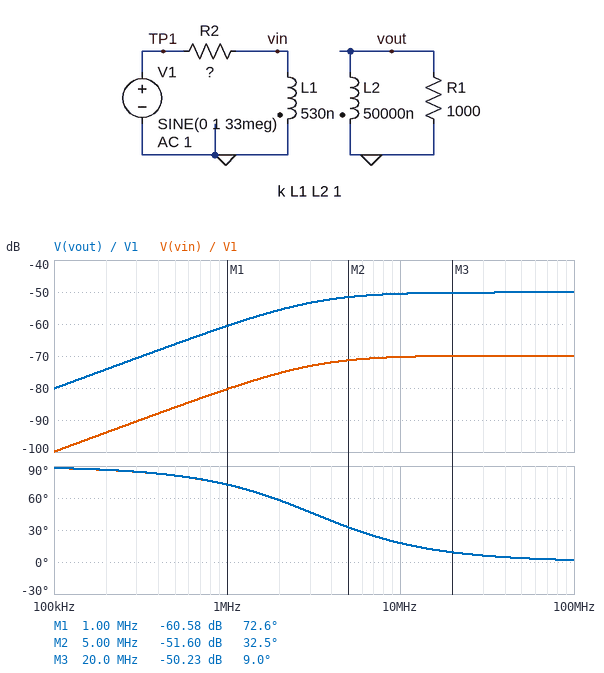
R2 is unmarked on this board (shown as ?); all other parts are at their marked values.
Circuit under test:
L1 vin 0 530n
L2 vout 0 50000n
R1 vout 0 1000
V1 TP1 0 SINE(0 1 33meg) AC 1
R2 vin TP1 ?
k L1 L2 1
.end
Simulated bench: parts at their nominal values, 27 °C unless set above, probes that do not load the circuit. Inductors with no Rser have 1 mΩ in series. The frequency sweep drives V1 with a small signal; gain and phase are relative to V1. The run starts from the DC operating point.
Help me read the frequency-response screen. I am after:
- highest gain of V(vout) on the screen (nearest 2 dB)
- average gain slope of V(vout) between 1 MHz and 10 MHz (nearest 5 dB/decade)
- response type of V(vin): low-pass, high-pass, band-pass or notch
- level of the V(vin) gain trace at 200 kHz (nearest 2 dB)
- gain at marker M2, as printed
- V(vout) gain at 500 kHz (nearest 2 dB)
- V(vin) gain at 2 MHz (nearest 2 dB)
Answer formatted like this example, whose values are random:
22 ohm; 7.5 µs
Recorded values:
-50 dB; 10 dB/decade; high-pass; -94 dB; -51.60 dB; -66 dB; -76 dB
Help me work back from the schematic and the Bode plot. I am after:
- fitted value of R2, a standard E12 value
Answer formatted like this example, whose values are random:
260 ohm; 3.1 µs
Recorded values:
33 kΩ
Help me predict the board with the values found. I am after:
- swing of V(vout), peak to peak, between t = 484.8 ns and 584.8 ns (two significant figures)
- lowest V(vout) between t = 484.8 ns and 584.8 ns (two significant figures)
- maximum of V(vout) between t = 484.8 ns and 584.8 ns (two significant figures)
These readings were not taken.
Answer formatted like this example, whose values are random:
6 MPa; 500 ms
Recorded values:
6.2 mV; -3.1 mV; 3.1 mV
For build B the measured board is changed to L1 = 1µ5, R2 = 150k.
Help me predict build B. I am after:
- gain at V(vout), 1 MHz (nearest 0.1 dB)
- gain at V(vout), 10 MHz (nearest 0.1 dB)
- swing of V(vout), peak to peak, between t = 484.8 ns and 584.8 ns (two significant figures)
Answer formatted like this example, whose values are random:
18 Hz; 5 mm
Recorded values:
-69.2 dB; -59.2 dB; 2.3 mV
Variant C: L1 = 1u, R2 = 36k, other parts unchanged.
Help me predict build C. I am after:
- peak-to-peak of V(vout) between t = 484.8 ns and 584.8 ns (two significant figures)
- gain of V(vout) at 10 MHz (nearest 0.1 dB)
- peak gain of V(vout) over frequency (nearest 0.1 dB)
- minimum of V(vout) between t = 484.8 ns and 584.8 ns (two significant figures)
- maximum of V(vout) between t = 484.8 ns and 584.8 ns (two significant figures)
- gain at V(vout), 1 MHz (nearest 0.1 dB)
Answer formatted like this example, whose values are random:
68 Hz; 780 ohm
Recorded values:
7.8 mV; -48.5 dB; -48.1 dB; -3.9 mV; 3.9 mV; -58.6 dB
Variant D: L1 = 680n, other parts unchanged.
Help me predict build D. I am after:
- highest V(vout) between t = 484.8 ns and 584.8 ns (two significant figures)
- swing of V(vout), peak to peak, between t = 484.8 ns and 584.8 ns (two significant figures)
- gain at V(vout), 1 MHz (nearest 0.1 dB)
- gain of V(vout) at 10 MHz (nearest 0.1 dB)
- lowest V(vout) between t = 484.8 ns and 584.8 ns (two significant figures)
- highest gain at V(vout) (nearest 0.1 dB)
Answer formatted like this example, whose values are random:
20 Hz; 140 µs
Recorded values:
3.5 mV; 7.0 mV; -59.5 dB; -49.5 dB; -3.5 mV; -49.0 dB
